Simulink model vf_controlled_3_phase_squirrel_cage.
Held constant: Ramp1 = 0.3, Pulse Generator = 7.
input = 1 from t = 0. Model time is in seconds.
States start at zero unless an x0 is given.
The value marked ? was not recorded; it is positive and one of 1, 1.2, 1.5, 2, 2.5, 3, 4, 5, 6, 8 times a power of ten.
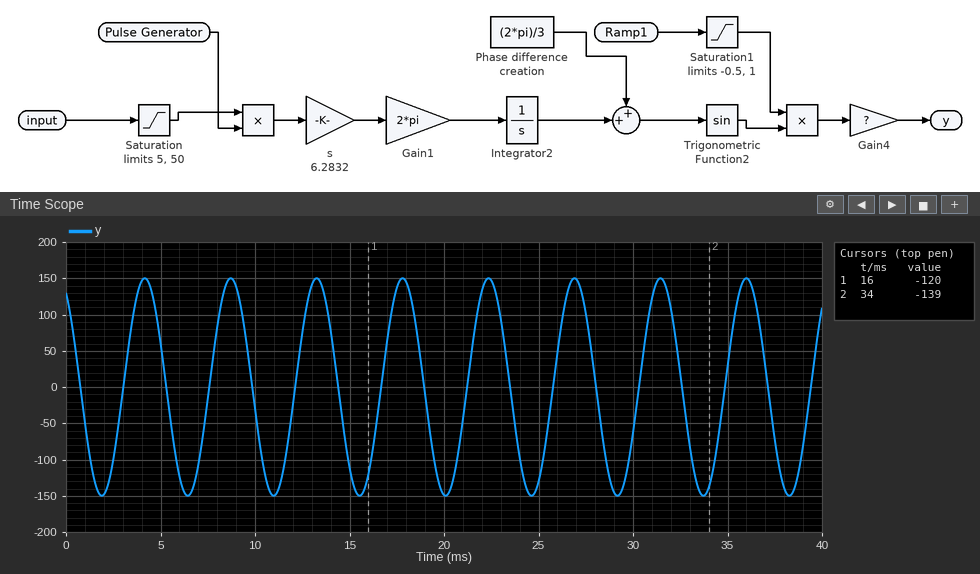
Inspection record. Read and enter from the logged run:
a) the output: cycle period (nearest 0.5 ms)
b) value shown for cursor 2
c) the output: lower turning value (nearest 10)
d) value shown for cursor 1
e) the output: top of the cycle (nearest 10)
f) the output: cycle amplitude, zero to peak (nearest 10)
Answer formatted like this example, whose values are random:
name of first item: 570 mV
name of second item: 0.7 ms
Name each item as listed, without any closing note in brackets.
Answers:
the output: cycle period: 4.5 ms
value shown for cursor 2: -139
the output: lower turning value: -150
value shown for cursor 1: -120
the output: top of the cycle: 150
the output: cycle amplitude, zero to peak: 150
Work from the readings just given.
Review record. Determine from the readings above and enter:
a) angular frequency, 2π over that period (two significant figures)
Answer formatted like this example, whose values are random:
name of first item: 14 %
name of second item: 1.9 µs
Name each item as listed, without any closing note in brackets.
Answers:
angular frequency, 2π over that period: 1.4 rad/ms
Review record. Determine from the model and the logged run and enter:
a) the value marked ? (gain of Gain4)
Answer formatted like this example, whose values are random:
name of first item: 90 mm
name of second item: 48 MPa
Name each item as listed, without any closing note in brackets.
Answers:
the value marked ?: 500
